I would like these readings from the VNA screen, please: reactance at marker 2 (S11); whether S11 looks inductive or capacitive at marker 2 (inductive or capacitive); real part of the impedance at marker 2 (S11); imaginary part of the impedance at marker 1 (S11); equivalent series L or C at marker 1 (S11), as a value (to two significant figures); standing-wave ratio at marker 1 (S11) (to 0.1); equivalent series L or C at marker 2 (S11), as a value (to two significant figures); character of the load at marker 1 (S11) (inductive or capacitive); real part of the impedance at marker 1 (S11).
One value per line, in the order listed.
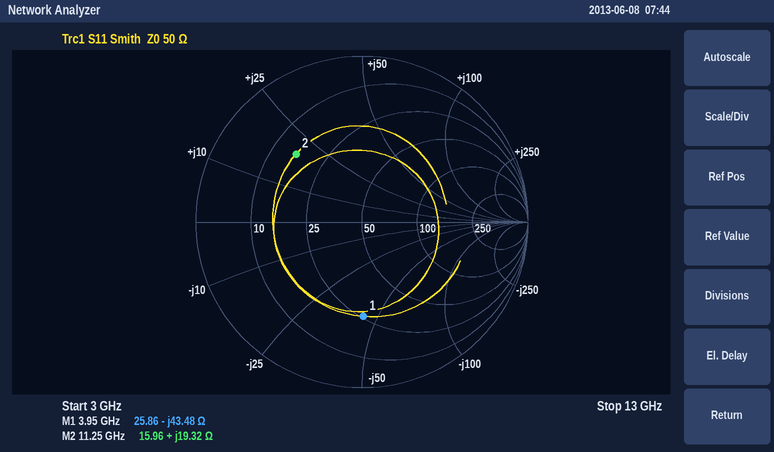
+19.32 Ω
inductive
15.96 Ω
-43.48 Ω
930 fF
3.6
270 pH
capacitive
25.86 Ω
